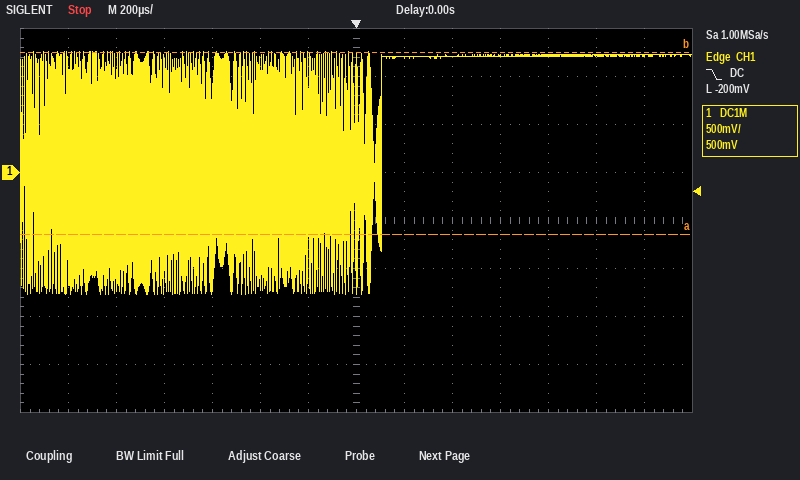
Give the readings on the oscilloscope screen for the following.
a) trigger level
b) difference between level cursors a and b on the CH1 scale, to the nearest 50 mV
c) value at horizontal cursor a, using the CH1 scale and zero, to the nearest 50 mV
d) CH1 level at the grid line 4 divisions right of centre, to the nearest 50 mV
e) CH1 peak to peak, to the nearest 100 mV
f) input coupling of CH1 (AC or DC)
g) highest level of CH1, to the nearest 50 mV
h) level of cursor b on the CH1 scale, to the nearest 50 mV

-200 mV
1.90 V
-650 mV
1.20 V
2.50 V
DC
1.25 V
1.25 V
